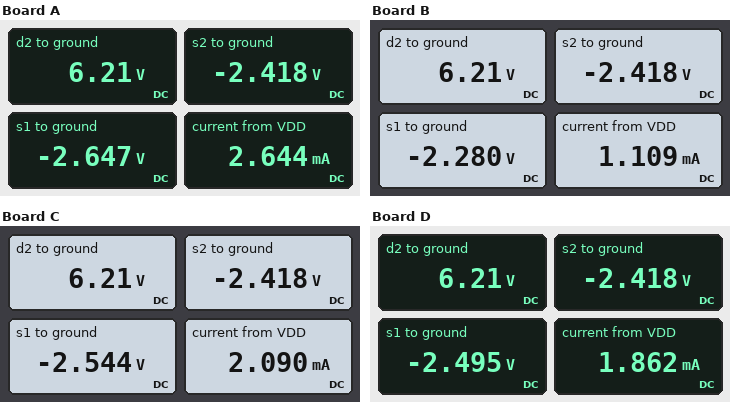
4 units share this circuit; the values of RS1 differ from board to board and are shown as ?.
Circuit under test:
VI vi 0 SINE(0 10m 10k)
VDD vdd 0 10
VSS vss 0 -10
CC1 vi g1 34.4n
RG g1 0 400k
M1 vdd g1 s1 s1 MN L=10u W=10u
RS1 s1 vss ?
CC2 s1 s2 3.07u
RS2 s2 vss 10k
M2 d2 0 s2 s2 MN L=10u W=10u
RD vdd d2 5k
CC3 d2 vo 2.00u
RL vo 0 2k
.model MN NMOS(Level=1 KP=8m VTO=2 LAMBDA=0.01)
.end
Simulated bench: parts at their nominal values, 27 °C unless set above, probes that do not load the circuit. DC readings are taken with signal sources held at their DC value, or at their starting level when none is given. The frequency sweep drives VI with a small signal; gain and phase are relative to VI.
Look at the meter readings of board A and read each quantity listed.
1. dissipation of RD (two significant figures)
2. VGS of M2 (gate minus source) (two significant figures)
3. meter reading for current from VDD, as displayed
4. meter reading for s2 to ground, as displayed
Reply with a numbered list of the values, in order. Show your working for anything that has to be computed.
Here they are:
1. (10 V - 6.21 V)^2 / 5 kΩ = 2.9 mW
2. 0 V - (-2.418 V) = 2.4 V
3. 2.644 mA
4. -2.418 V
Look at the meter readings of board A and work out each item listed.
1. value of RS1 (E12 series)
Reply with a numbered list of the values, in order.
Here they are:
1. 3.9 kΩ
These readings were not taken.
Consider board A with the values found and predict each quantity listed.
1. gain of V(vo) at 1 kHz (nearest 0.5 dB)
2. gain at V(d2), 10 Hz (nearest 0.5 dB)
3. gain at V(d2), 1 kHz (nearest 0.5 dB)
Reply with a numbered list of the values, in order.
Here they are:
1. 9.5 dB
2. -7.0 dB
3. 9.5 dB
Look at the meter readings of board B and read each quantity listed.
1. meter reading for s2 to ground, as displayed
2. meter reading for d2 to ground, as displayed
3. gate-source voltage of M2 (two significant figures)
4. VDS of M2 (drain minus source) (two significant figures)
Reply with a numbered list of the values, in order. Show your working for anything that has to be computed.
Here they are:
1. -2.418 V
2. 6.21 V
3. 0 V - (-2.418 V) = 2.4 V
4. 6.21 V - (-2.418 V) = 8.6 V
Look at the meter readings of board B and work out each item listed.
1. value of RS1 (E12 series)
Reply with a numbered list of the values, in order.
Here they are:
1. 22 kΩ
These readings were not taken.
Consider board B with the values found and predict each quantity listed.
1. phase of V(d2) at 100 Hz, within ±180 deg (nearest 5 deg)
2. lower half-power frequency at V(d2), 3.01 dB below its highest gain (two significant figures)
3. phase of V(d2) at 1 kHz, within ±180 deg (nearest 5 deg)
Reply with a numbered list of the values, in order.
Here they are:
1. 30 deg
2. 61 Hz
3. 5 deg
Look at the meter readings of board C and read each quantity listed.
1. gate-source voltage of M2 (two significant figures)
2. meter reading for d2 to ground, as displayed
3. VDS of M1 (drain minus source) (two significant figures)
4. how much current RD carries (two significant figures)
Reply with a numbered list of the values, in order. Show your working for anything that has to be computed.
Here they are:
1. 0 V - (-2.418 V) = 2.4 V
2. 6.21 V
3. 10 V - (-2.544 V) = 13 V
4. (10 V - 6.21 V) / 5 kΩ = 760 µA
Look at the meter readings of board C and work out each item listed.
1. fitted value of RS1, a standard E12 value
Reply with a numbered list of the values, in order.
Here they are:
1. 5.6 kΩ
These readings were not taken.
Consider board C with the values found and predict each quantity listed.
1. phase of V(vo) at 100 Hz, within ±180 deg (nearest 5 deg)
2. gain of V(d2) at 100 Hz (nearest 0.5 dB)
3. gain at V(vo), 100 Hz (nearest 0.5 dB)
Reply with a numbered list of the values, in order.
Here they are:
1. 60 deg
2. 6.0 dB
3. 5.5 dB
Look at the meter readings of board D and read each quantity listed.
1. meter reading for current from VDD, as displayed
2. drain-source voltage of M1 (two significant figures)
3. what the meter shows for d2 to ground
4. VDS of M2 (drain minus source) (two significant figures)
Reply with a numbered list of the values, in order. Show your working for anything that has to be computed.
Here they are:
1. 1.862 mA
2. 10 V - (-2.495 V) = 12 V
3. 6.21 V
4. 6.21 V - (-2.418 V) = 8.6 V
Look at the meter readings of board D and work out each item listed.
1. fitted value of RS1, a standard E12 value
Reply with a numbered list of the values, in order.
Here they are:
1. 6.8 kΩ
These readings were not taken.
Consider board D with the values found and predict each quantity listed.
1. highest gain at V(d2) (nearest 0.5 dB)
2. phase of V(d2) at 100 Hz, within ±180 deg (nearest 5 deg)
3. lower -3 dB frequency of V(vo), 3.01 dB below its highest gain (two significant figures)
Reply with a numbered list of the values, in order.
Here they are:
1. 9.0 dB
2. 40 deg
3. 110 Hz
